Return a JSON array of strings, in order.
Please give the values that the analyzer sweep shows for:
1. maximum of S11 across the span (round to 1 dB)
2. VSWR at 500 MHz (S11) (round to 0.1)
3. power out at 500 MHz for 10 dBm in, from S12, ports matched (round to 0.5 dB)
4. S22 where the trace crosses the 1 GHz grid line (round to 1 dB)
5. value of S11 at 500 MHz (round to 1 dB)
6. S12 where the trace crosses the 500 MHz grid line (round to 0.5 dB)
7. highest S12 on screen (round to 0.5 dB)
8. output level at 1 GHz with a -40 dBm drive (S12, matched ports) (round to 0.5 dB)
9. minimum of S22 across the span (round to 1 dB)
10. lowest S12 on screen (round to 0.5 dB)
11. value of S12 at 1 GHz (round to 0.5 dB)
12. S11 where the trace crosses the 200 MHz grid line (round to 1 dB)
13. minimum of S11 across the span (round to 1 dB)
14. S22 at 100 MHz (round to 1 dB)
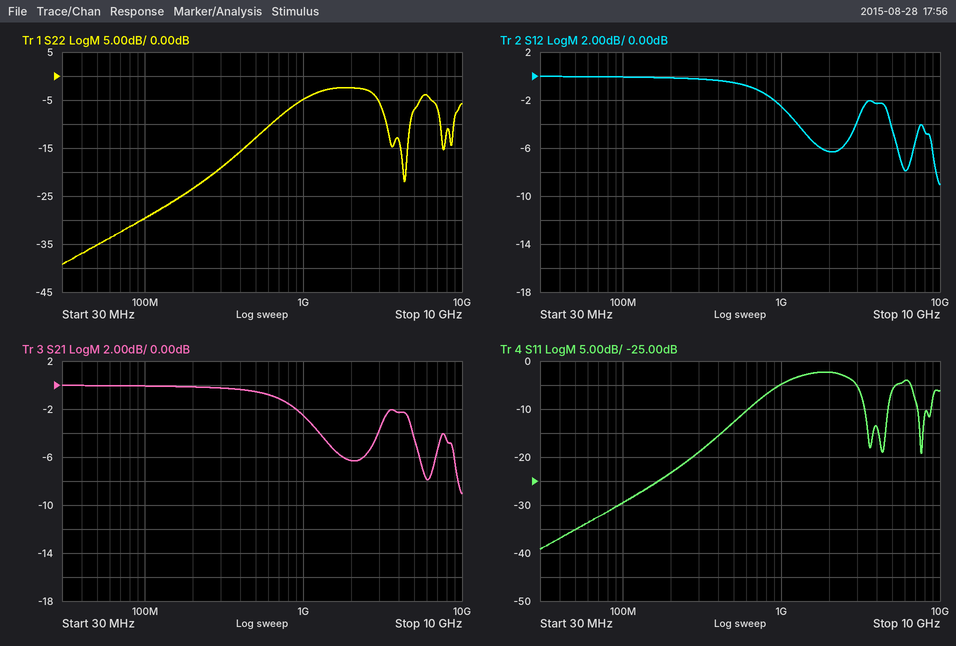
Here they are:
["-2 dB", "1.6", "9.5 dBm", "-5 dB", "-13 dB", "-0.5 dB", "0.0 dB", "-42.5 dBm", "-39 dB", "-9.0 dB", "-2.5 dB", "-23 dB", "-39 dB", "-30 dB"]
